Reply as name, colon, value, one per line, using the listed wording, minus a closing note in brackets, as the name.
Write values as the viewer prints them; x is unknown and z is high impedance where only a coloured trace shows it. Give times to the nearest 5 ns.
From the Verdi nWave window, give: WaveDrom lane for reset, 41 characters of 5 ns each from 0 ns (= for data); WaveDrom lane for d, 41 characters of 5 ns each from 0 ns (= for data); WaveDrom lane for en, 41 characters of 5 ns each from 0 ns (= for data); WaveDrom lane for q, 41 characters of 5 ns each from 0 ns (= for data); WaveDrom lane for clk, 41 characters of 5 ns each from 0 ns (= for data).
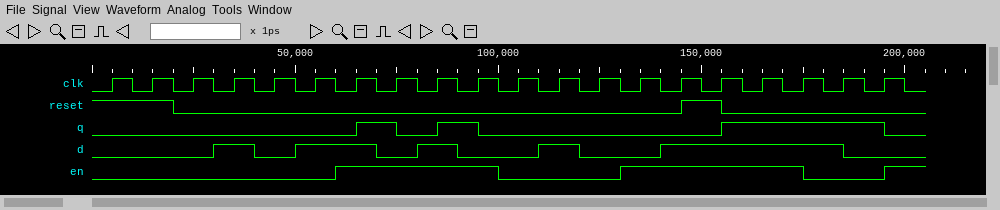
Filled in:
WaveDrom lane for reset, 41 characters of 5 ns each from 0 ns: {name: 'reset', wave: '1...0........................1.0.........'}
WaveDrom lane for d, 41 characters of 5 ns each from 0 ns: {name: 'd', wave: '0.....1.0.1...0.1.0...1.0...1........0...'}
WaveDrom lane for en, 41 characters of 5 ns each from 0 ns: {name: 'en', wave: '0...........1.......0.....1........0...1.'}
WaveDrom lane for q, 41 characters of 5 ns each from 0 ns: {name: 'q', wave: '0............1.0.1.0...........1.......0.'}
WaveDrom lane for clk, 41 characters of 5 ns each from 0 ns: {name: 'clk', wave: '01010101010101010101010101010101010101010'}
